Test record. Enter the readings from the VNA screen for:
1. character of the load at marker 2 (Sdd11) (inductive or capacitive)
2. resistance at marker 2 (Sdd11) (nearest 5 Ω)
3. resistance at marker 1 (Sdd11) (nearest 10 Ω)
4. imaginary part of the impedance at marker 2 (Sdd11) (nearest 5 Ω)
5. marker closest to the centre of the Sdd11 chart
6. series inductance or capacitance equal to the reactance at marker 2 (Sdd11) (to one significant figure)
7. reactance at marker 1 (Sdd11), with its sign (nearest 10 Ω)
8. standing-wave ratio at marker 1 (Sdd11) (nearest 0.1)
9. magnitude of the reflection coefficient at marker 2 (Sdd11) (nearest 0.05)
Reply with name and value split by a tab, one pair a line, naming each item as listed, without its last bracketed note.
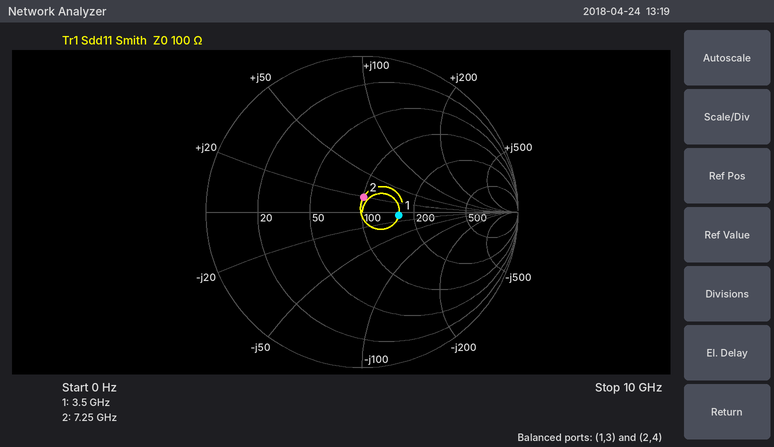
character of the load at marker 2 (Sdd11)	inductive
resistance at marker 2 (Sdd11)	100 Ω
resistance at marker 1 (Sdd11)	160 Ω
imaginary part of the impedance at marker 2 (Sdd11)	+20 Ω
marker closest to the centre of the Sdd11 chart	marker 2
series inductance or capacitance equal to the reactance at marker 2 (Sdd11)	400 pH
reactance at marker 1 (Sdd11), with its sign	-10 Ω
standing-wave ratio at marker 1 (Sdd11)	1.6
magnitude of the reflection coefficient at marker 2 (Sdd11)	0.10
